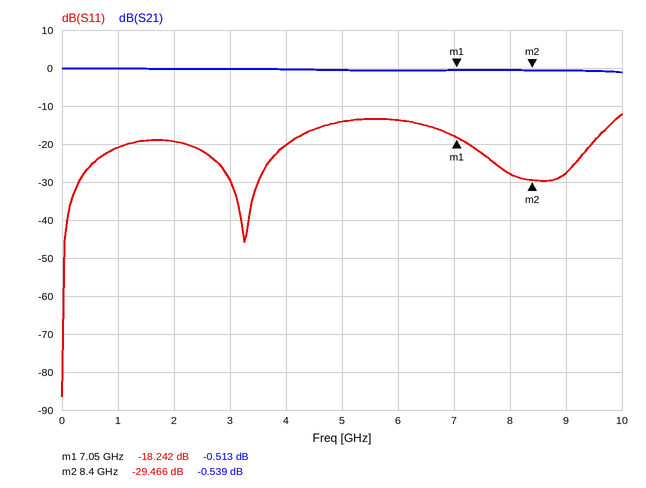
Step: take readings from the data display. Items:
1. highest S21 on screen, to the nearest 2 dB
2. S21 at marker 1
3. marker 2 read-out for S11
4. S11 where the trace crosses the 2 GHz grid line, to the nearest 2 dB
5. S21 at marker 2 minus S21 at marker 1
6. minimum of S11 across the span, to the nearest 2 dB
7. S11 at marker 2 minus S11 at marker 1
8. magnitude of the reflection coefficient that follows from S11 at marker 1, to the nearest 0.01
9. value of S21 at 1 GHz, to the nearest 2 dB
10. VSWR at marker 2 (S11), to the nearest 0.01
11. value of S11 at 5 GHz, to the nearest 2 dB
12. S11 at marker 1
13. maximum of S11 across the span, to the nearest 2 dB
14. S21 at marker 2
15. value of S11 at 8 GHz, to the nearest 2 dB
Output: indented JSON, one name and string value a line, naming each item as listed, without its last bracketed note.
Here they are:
{
  "highest S21 on screen, to the nearest 2 dB": "0 dB",
  "S21 at marker 1": "-0.513 dB",
  "marker 2 read-out for S11": "-29.466 dB",
  "S11 where the trace crosses the 2 GHz grid line, to the nearest 2 dB": "-20 dB",
  "S21 at marker 2 minus S21 at marker 1": "-0.026 dB",
  "minimum of S11 across the span, to the nearest 2 dB": "-86 dB",
  "S11 at marker 2 minus S11 at marker 1": "-11.224 dB",
  "magnitude of the reflection coefficient that follows from S11 at marker 1, to the nearest 0.01": "0.12",
  "value of S21 at 1 GHz, to the nearest 2 dB": "0 dB",
  "VSWR at marker 2 (S11), to the nearest 0.01": "1.07",
  "value of S11 at 5 GHz, to the nearest 2 dB": "-14 dB",
  "S11 at marker 1": "-18.242 dB",
  "maximum of S11 across the span, to the nearest 2 dB": "-12 dB",
  "S21 at marker 2": "-0.539 dB",
  "value of S11 at 8 GHz, to the nearest 2 dB": "-28 dB"
}
